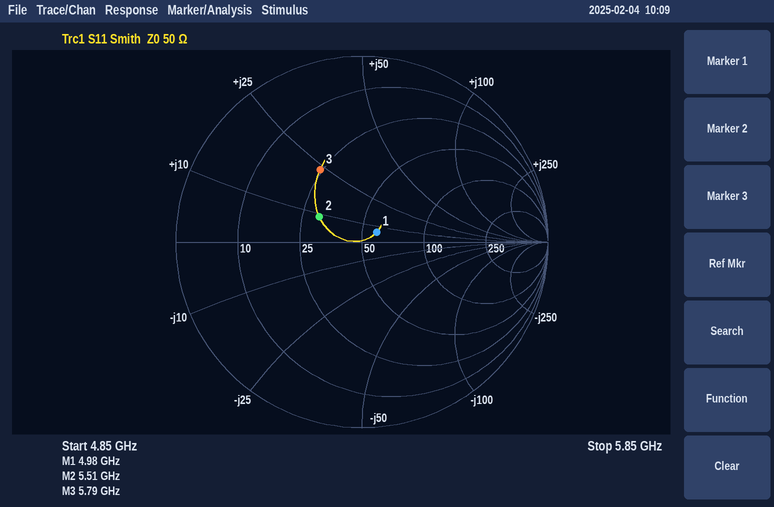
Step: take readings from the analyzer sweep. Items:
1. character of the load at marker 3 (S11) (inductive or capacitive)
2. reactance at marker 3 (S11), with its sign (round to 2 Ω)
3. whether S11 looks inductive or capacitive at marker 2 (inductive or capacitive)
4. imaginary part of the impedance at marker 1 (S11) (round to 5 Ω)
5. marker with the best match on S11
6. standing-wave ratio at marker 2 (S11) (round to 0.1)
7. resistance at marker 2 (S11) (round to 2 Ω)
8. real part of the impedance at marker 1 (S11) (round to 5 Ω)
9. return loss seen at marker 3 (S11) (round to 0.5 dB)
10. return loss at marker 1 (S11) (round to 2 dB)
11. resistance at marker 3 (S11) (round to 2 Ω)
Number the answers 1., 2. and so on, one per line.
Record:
1. inductive
2. +24 Ω
3. inductive
4. +5 Ω
5. marker 1
6. 1.7
7. 30 Ω
8. 60 Ω
9. 7.0 dB
10. 20 dB
11. 24 Ω
